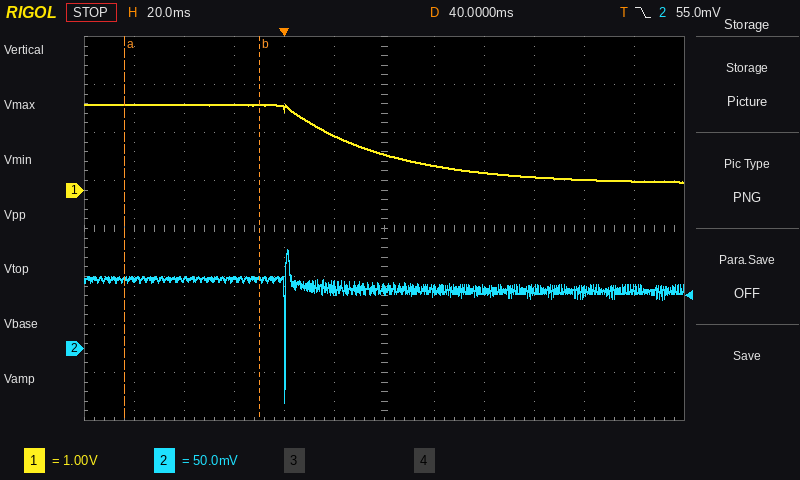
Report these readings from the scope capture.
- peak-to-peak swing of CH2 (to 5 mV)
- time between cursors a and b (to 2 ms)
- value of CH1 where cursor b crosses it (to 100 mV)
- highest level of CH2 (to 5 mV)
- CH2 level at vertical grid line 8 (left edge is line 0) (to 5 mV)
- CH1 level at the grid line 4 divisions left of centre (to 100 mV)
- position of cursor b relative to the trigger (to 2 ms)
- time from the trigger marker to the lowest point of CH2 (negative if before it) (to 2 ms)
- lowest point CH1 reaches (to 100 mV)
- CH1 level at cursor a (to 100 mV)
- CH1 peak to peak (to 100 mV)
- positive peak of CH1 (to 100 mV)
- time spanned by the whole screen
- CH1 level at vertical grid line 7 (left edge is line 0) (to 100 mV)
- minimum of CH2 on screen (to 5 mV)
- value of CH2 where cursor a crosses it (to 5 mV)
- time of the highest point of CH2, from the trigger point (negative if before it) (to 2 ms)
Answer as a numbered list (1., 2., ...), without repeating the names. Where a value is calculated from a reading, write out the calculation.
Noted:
1. 105 mV − (-55 mV) = 160 mV
2. 54 ms
3. 1.8 V
4. 105 mV
5. 60 mV
6. 1.8 V
7. -10 ms
8. 0 ms
9. 200 mV
10. 1.8 V
11. 1.8 V − (200 mV) = 1.6 V
12. 1.8 V
13. 240 ms
14. 500 mV
15. -55 mV
16. 70 mV
17. +2 ms
